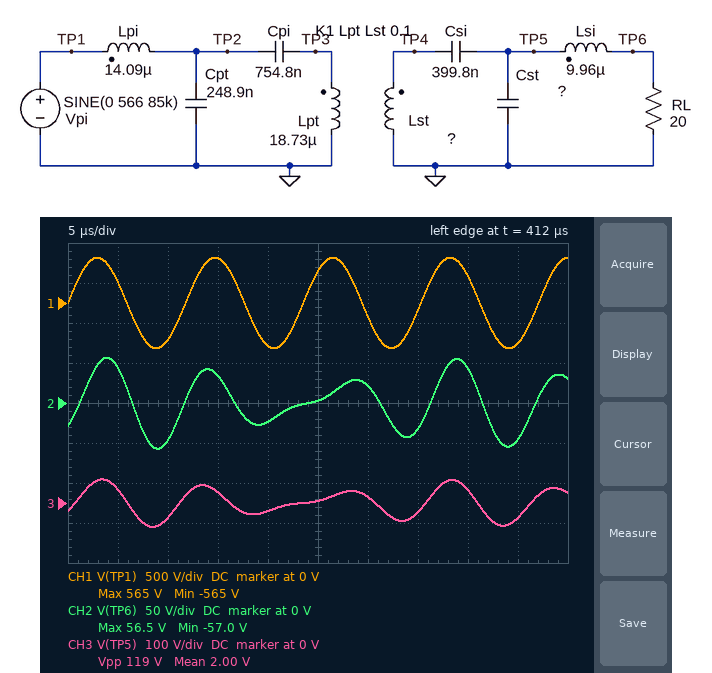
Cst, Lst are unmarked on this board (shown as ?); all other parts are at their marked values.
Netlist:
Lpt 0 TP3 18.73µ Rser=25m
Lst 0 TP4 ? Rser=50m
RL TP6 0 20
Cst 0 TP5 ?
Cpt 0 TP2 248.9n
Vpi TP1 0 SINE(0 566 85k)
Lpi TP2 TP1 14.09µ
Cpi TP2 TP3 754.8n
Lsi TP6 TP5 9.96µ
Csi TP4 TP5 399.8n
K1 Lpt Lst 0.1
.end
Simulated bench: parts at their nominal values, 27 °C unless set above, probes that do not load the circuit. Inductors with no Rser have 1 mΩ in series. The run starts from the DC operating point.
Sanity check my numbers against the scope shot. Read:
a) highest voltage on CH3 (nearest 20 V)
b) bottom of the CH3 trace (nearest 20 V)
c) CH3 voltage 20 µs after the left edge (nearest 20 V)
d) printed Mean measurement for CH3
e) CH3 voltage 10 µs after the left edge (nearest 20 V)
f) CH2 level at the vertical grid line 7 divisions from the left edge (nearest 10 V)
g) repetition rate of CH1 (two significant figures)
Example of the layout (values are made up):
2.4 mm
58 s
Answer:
60 V
-60 V
-20 V
2.00 V
-40 V
-30 V
85 kHz
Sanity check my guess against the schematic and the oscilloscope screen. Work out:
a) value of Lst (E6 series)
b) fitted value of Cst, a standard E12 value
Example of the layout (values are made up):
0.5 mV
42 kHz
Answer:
6.8 µH
560 nF
